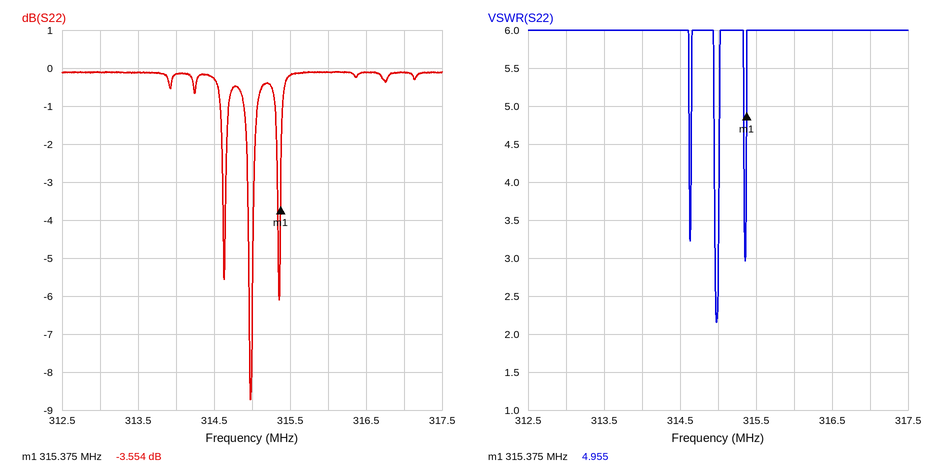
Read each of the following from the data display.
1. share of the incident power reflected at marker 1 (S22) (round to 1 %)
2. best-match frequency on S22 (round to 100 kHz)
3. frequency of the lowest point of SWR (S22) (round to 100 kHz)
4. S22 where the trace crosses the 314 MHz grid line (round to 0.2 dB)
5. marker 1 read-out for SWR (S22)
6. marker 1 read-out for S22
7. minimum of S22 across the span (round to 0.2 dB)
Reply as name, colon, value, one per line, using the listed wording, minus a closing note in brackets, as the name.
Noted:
share of the incident power reflected at marker 1 (S22): 44 %
best-match frequency on S22: 315.0 MHz
frequency of the lowest point of SWR (S22): 315.0 MHz
S22 where the trace crosses the 314 MHz grid line: -0.2 dB
marker 1 read-out for SWR: 4.955
marker 1 read-out for S22: -3.554 dB
minimum of S22 across the span: -8.8 dB
